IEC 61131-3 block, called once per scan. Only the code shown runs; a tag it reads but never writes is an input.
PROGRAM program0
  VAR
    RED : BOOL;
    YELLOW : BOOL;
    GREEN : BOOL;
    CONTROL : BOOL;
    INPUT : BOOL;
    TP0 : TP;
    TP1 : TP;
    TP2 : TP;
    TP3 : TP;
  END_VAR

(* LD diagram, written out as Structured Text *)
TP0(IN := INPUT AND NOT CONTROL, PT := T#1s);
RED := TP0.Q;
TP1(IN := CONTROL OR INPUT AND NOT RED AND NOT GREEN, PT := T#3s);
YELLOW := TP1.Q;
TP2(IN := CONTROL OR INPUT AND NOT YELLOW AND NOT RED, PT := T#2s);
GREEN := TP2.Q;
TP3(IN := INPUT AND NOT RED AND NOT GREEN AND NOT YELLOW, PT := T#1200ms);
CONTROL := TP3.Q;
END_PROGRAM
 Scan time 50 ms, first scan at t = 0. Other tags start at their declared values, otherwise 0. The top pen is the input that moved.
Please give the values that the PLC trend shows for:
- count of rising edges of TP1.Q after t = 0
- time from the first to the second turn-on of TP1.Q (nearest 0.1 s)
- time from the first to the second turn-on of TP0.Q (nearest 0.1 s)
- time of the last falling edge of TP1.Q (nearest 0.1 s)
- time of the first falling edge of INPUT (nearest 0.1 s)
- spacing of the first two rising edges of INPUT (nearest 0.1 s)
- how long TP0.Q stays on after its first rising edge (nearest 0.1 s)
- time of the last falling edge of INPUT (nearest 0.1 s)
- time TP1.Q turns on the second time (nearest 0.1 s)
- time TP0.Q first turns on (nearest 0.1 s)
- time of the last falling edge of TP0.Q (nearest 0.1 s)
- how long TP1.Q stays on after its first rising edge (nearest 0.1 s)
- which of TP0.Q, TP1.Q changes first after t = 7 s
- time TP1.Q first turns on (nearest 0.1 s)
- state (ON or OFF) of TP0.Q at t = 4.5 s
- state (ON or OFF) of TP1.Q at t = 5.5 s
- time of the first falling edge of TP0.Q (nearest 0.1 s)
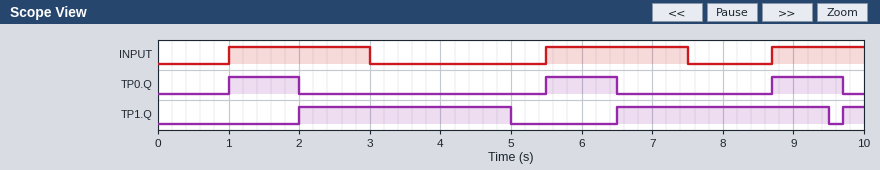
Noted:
3
4.5 s
4.5 s
9.5 s
3.0 s
4.5 s
1.0 s
7.5 s
6.5 s
1.0 s
9.7 s
3.0 s
TP0.Q
2.0 s
OFF
OFF
2.0 s
